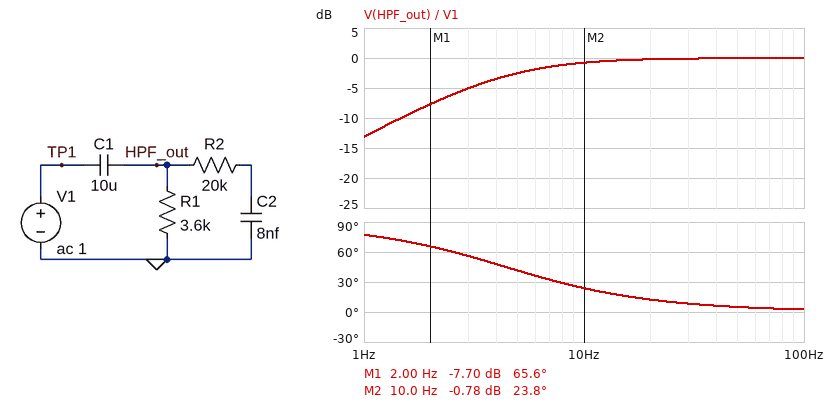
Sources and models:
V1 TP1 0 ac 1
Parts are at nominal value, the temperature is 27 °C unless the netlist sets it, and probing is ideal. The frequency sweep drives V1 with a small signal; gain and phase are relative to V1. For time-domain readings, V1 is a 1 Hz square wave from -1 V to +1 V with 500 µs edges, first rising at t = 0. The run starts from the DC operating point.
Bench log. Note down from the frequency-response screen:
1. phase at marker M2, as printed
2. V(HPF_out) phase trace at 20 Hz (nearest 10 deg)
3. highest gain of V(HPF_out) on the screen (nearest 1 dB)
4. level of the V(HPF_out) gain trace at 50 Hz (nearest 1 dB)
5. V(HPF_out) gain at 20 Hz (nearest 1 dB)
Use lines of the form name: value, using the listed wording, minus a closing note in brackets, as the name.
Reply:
phase at marker M2, as printed: 23.8 deg
V(HPF_out) phase trace at 20 Hz: 10 deg
highest gain of V(HPF_out) on the screen: 0 dB
level of the V(HPF_out) gain trace at 50 Hz: 0 dB
V(HPF_out) gain at 20 Hz: 0 dB
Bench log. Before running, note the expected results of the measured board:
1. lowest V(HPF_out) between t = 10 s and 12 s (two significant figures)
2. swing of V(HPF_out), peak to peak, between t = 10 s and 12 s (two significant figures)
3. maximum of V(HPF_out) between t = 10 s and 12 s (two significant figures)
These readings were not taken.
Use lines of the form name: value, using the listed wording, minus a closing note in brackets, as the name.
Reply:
lowest V(HPF_out) between t = 10 s and 12 s: -2.0 V
swing of V(HPF_out), peak to peak, between t = 10 s and 12 s: 4.0 V
maximum of V(HPF_out) between t = 10 s and 12 s: 2.0 V
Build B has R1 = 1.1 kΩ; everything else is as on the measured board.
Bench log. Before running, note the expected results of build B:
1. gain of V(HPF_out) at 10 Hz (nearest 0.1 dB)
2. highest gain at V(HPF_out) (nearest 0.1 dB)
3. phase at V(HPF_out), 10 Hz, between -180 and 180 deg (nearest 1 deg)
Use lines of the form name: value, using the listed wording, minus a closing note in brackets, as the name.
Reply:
gain of V(HPF_out) at 10 Hz: -4.9 dB
highest gain at V(HPF_out): 0 dB
phase at V(HPF_out), 10 Hz, between -180 and 180 deg: 55 deg
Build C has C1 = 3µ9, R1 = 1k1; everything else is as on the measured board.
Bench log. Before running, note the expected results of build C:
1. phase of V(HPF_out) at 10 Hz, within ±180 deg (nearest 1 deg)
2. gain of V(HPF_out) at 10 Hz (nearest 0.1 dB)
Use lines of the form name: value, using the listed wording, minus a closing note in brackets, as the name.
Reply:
phase of V(HPF_out) at 10 Hz, within ±180 deg: 75 deg
gain of V(HPF_out) at 10 Hz: -11.7 dB
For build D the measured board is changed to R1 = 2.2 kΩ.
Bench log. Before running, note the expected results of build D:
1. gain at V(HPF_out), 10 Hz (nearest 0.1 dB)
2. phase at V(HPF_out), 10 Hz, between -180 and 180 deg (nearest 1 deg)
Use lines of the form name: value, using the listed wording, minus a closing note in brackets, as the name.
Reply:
gain at V(HPF_out), 10 Hz: -1.8 dB
phase at V(HPF_out), 10 Hz, between -180 and 180 deg: 36 deg
